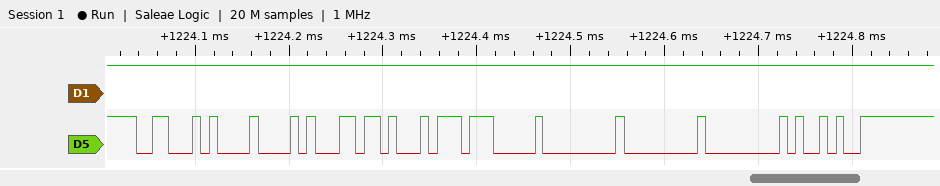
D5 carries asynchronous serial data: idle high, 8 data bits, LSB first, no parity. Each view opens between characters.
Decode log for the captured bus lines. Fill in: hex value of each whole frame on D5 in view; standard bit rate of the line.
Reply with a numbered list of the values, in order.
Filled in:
1. 46, 08, B1, D1, 07, 00, 00, 00, 29
2. 115200 baud
